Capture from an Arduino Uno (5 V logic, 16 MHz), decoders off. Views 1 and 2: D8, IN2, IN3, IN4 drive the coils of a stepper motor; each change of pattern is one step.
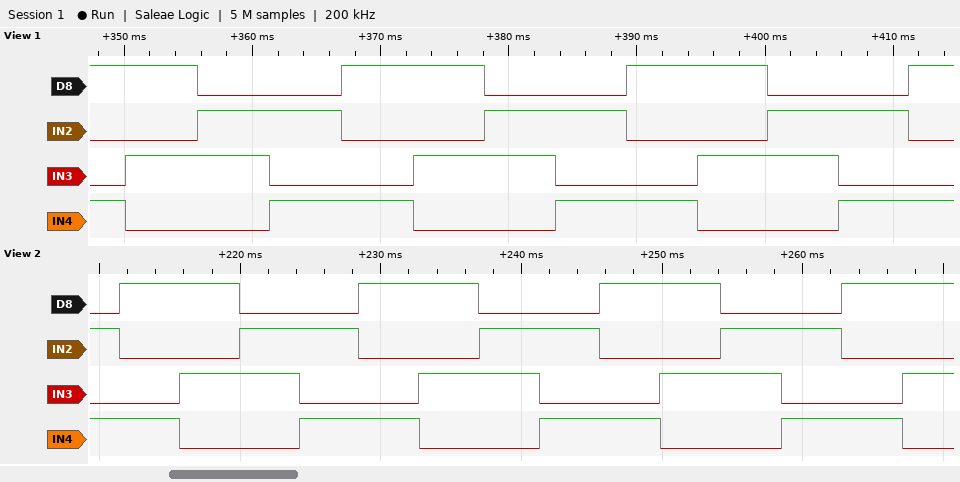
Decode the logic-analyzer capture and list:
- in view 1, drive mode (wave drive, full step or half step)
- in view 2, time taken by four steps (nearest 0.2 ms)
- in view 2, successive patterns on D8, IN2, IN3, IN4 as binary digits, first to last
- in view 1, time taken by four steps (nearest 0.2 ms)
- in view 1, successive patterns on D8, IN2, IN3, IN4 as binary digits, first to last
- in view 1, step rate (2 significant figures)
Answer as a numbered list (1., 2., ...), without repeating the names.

1. full step
2. 17.0 ms
3. 0101 1001 1010 0110 0101 1001 1010 0110 0101 1001 1010 0110 0101 1001 1010
4. 22.4 ms
5. 1001 1010 0110 0101 1001 1010 0110 0101 1001 1010 0110 0101 1001
6. 180 steps/s
